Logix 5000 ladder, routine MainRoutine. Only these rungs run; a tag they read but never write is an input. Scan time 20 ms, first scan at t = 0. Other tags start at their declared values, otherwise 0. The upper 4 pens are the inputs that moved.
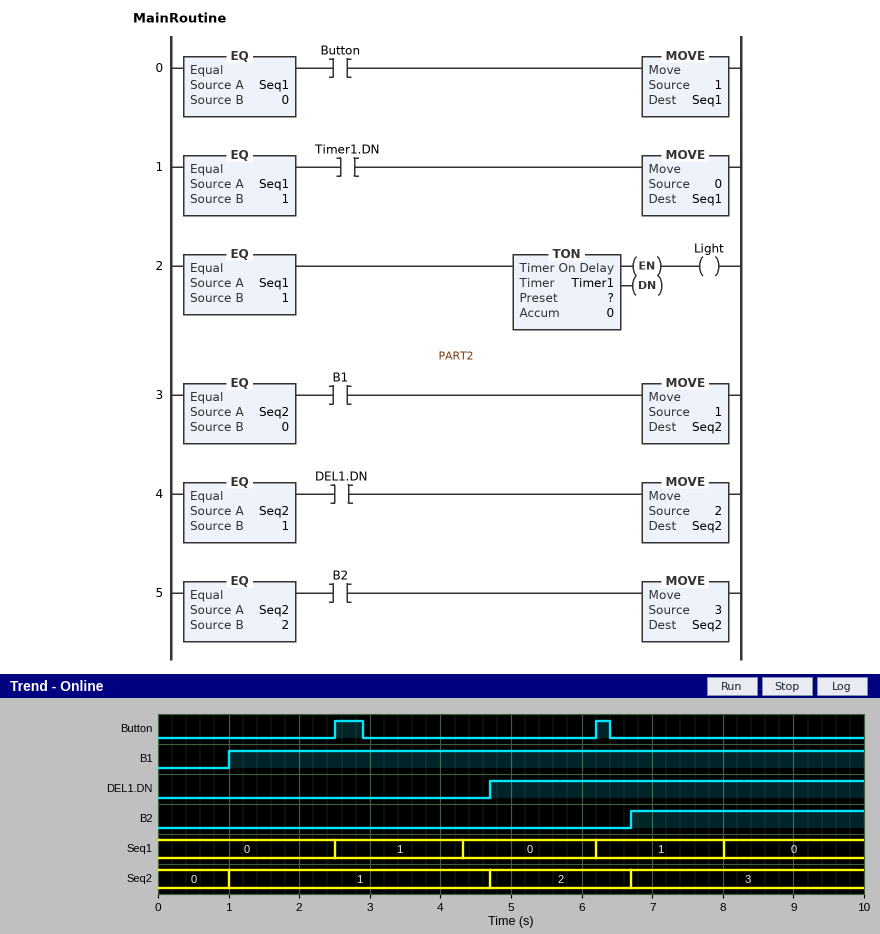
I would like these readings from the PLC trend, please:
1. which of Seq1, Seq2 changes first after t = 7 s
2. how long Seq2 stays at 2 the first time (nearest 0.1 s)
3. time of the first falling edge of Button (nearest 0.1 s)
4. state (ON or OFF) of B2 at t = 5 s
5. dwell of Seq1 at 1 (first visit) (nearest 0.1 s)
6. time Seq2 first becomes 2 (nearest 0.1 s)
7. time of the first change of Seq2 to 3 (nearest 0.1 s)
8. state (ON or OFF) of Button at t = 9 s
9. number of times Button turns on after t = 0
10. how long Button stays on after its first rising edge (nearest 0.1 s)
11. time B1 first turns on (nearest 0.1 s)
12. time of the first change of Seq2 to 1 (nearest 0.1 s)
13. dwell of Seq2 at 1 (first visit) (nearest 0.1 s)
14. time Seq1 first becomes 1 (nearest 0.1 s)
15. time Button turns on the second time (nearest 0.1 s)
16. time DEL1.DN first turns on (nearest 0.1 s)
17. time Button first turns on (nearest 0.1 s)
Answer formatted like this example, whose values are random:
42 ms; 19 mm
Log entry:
Seq1; 2.0 s; 2.9 s; OFF; 1.8 s; 4.7 s; 6.7 s; OFF; 2; 0.4 s; 1.0 s; 1.0 s; 3.7 s; 2.5 s; 6.2 s; 4.7 s; 2.5 s
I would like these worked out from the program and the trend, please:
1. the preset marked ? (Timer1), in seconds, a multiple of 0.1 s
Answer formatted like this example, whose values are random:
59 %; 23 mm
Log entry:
1.8 s
